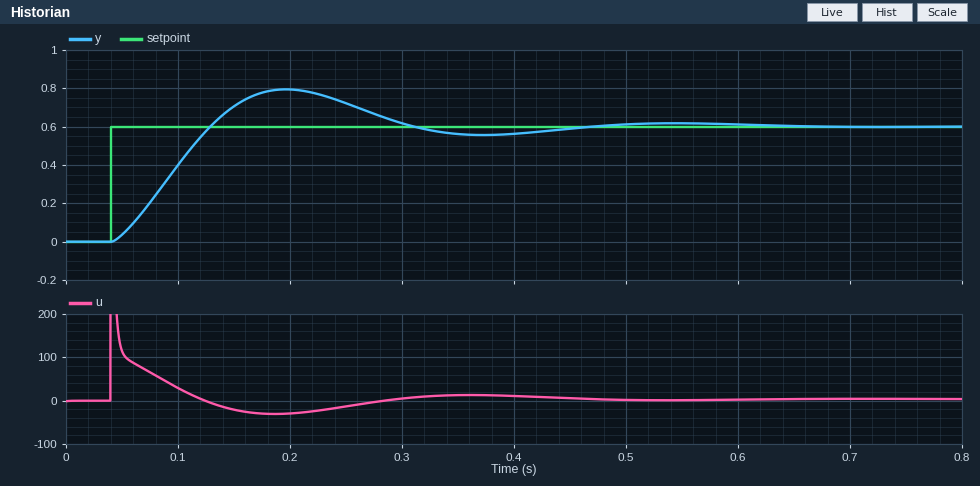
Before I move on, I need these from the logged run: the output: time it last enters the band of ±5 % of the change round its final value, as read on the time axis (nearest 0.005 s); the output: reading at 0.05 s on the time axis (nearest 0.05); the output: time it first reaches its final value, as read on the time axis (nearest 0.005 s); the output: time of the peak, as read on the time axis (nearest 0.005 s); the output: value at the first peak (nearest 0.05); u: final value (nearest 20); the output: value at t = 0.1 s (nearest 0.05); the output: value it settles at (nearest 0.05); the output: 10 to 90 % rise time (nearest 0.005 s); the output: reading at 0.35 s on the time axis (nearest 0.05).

0.415 s
0.05
0.130 s
0.195 s
0.80
0
0.40
0.60
0.065 s
0.55
